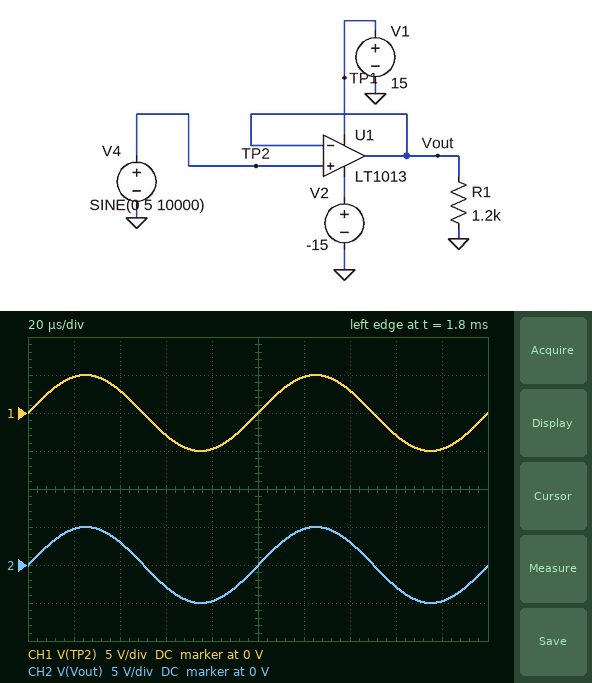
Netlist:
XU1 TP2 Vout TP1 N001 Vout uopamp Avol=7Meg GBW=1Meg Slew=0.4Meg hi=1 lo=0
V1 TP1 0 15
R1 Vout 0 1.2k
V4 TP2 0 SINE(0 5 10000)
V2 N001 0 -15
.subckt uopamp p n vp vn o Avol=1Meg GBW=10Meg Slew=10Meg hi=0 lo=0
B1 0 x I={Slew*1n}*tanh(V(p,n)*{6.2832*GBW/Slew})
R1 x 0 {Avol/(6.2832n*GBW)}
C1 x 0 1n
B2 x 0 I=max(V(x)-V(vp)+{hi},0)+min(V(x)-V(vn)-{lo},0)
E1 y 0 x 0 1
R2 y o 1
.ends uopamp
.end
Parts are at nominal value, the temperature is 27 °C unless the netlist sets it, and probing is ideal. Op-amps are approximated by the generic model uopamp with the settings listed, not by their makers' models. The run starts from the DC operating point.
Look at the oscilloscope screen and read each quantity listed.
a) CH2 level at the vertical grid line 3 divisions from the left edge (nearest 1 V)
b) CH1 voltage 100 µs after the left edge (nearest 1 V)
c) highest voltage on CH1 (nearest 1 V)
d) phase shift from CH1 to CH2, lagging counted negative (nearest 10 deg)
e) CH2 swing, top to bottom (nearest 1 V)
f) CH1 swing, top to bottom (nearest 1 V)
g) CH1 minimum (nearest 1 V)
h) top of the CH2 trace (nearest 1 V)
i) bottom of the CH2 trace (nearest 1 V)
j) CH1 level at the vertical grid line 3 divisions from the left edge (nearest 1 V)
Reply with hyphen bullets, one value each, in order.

- -3 V
- 0 V
- 5 V
- 0 deg
- 10 V
- 10 V
- -5 V
- 5 V
- -5 V
- -3 V
